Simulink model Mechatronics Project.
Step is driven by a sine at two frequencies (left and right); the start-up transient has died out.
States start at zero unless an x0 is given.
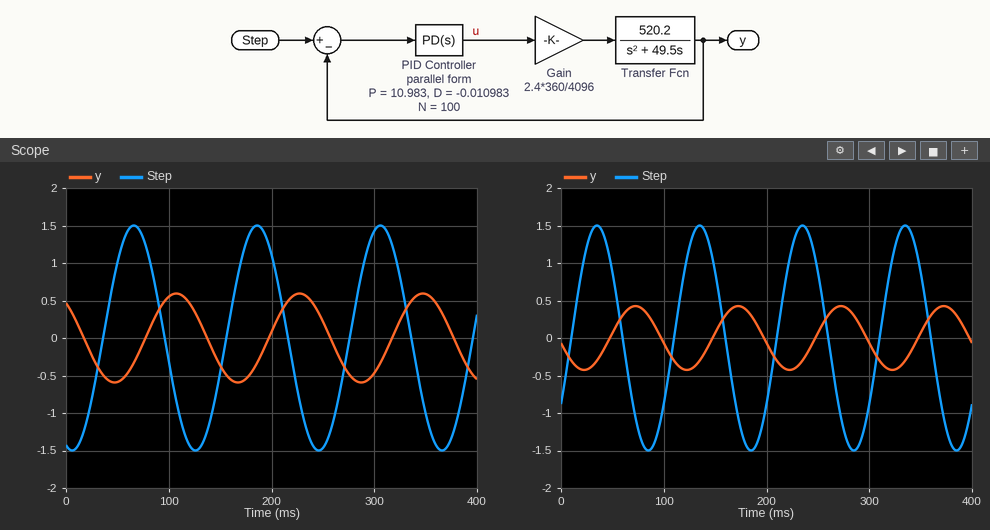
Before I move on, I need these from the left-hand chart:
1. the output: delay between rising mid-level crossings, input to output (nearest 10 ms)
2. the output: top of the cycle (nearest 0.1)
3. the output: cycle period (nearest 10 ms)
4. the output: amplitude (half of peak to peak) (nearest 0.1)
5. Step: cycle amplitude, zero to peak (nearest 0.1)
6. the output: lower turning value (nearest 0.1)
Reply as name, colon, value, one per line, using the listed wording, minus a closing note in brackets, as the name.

the output: delay between rising mid-level crossings, input to output: 40 ms
the output: top of the cycle: 0.6
the output: cycle period: 120 ms
the output: amplitude (half of peak to peak): 0.6
Step: cycle amplitude, zero to peak: 1.5
the output: lower turning value: -0.6
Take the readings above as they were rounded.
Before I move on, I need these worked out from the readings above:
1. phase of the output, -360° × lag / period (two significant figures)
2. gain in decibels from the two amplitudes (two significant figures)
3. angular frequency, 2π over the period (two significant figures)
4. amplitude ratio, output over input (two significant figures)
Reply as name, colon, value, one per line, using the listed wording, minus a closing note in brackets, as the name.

phase of the output, -360° × lag / period: -120°
gain in decibels from the two amplitudes: -8.0 dB
angular frequency, 2π over the period: 0.052 rad/ms
amplitude ratio, output over input: 0.40
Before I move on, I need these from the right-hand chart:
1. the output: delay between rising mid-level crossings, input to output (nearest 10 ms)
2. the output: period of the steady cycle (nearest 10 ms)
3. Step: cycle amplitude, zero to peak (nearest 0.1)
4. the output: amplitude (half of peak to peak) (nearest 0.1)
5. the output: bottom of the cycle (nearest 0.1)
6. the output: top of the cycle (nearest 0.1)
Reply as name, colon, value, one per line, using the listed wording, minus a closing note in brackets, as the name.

the output: delay between rising mid-level crossings, input to output: 40 ms
the output: period of the steady cycle: 100 ms
Step: cycle amplitude, zero to peak: 1.5
the output: amplitude (half of peak to peak): 0.4
the output: bottom of the cycle: -0.4
the output: top of the cycle: 0.4
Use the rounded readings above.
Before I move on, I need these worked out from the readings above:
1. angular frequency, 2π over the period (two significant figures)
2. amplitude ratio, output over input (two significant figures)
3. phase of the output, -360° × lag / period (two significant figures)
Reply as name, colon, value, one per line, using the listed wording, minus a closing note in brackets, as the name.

angular frequency, 2π over the period: 0.063 rad/ms
amplitude ratio, output over input: 0.27
phase of the output, -360° × lag / period: -140°
